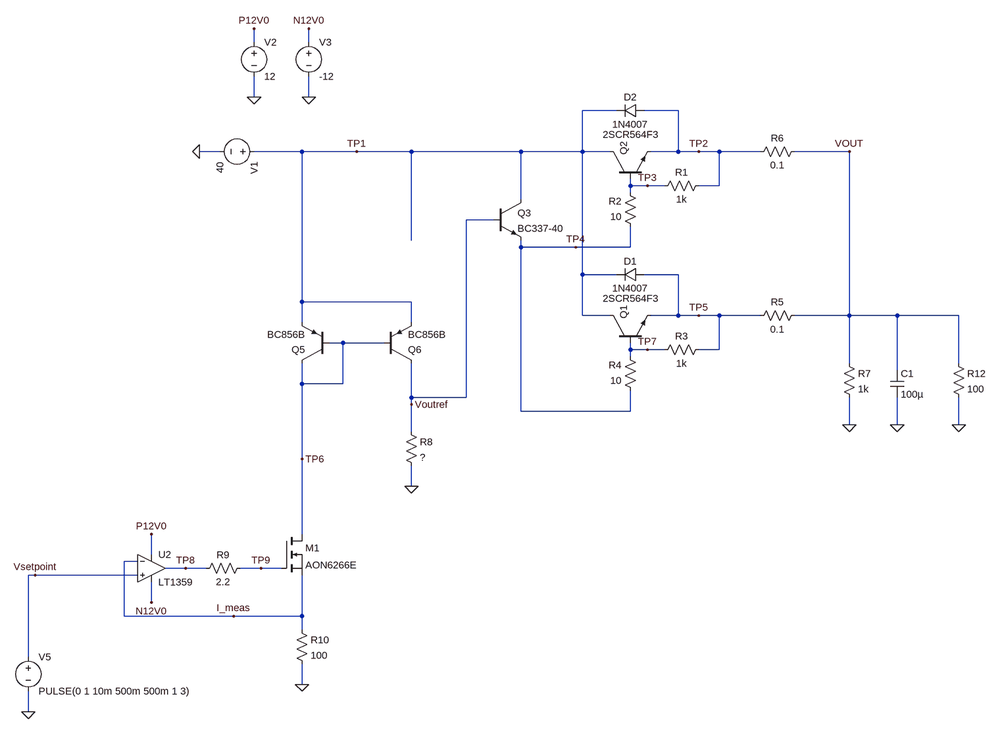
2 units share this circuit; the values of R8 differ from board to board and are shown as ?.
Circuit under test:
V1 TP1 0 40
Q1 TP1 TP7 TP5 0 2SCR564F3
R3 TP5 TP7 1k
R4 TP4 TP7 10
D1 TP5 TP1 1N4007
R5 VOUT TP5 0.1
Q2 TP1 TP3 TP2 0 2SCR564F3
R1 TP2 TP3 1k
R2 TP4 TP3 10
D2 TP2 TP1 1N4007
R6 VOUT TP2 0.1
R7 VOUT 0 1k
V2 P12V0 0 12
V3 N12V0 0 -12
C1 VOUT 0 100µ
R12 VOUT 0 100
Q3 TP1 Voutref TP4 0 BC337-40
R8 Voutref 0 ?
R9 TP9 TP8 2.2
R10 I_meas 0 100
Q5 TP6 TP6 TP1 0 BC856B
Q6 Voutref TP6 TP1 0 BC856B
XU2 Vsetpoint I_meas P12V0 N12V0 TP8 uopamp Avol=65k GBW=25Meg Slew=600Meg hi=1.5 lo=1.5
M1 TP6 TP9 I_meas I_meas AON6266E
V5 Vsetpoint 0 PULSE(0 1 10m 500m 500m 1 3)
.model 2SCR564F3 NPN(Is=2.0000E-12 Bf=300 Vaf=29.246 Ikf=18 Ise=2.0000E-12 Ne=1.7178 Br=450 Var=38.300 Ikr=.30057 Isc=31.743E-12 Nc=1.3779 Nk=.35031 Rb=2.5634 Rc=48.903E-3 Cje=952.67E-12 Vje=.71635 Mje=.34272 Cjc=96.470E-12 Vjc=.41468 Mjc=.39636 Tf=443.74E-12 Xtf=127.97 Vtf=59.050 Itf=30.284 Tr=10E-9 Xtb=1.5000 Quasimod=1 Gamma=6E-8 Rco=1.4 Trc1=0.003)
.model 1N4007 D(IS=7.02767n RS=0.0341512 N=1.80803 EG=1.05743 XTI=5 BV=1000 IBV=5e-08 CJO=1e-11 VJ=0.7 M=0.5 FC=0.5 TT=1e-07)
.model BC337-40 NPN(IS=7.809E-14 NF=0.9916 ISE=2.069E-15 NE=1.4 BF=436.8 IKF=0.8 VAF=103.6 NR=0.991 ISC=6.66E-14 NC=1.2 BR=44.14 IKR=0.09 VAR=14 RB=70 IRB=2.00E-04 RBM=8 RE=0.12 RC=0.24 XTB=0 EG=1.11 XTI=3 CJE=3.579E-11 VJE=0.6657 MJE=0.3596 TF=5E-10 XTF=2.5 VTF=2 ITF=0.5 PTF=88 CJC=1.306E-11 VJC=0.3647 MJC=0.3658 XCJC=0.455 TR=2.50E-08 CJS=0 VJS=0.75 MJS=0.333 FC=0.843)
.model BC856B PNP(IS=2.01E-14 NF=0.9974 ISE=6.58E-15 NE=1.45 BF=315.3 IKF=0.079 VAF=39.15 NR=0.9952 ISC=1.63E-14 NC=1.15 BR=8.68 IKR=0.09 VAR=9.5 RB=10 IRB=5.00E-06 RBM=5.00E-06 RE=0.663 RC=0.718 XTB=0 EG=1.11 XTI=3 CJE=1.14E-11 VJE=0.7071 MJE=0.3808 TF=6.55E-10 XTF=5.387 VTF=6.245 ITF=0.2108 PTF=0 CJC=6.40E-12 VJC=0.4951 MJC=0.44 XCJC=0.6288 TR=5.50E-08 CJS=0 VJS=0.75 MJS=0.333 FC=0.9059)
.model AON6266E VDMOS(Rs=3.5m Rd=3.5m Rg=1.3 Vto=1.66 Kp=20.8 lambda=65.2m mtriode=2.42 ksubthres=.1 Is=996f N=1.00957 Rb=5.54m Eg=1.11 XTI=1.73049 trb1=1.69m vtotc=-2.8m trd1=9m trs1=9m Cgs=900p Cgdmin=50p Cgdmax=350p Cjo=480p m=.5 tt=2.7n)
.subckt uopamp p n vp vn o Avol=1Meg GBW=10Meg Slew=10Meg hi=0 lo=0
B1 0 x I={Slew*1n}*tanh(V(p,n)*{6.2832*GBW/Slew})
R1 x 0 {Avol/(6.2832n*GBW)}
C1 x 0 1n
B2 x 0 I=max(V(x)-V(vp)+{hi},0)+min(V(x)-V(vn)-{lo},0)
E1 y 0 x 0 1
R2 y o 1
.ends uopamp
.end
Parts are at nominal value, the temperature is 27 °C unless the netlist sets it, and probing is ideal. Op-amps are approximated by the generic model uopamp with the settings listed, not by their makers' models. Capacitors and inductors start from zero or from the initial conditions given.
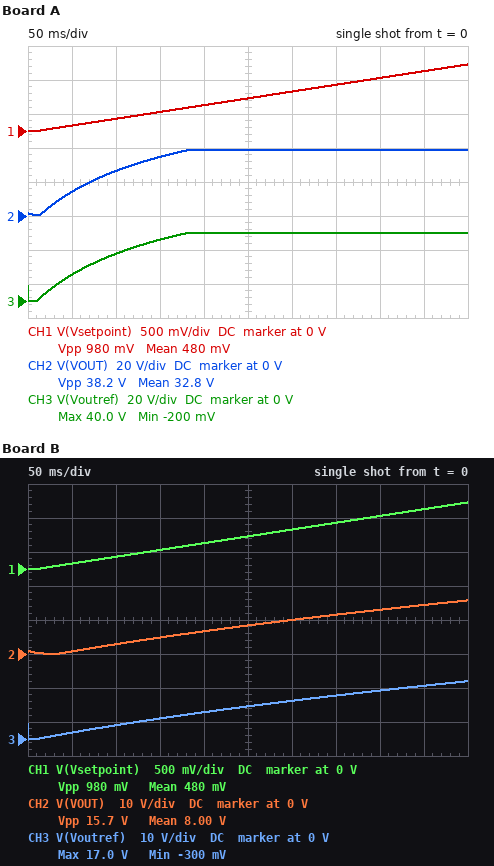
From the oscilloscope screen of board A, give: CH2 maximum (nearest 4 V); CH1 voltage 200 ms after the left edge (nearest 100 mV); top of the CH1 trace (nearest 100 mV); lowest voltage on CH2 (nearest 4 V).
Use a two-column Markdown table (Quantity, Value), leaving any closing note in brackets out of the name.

| Quantity | Value |
|---|---|
| CH2 maximum | 40 V |
| CH1 voltage 200 ms after the left edge | 400 mV |
| top of the CH1 trace | 1.0 V |
| lowest voltage on CH2 | 0 V |
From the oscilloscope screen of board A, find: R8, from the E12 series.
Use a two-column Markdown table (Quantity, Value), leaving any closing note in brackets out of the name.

| Quantity | Value |
|---|---|
| R8, from the E12 series | 12 kΩ |
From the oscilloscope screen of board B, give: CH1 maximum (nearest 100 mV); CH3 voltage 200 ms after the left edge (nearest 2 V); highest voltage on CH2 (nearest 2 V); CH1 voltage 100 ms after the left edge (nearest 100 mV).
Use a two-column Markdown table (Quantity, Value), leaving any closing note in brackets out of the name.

| Quantity | Value |
|---|---|
| CH1 maximum | 1.0 V |
| CH3 voltage 200 ms after the left edge | 8 V |
| highest voltage on CH2 | 16 V |
| CH1 voltage 100 ms after the left edge | 200 mV |
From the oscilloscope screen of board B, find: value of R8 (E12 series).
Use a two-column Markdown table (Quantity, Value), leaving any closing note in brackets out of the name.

| Quantity | Value |
|---|---|
| value of R8 | 1.2 kΩ |
